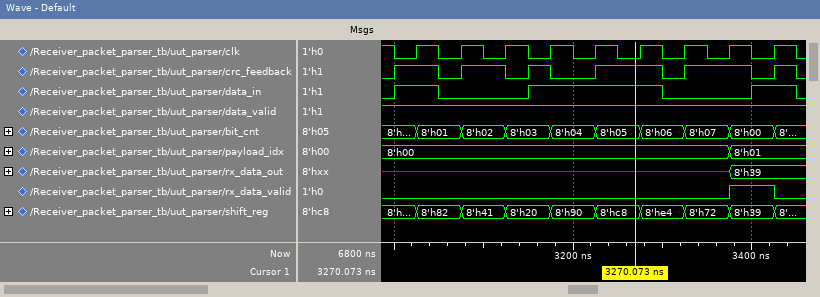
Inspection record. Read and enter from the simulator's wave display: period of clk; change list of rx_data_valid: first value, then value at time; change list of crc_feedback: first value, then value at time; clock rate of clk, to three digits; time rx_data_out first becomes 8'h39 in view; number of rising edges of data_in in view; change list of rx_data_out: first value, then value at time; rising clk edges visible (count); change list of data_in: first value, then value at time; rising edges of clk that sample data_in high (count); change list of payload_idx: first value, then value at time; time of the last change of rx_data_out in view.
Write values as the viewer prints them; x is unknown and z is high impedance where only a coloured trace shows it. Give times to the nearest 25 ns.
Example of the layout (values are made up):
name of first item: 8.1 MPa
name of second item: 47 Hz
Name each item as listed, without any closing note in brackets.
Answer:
period of clk: 50 ns
change list of rx_data_valid: first value, then value at time: 0, 1 at 3375 ns, 0 at 3425 ns
change list of crc_feedback: first value, then value at time: 0, 1 at 3000 ns, 0 at 3050 ns, 1 at 3075 ns, 0 at 3125 ns, 1 at 3150 ns, 0 at 3175 ns, 1 at 3225 ns, 0 at 3300 ns, 1 at 3325 ns, 0 at 3400 ns, 1 at 3425 ns, 0 at 3450 ns
clock rate of clk, to three digits: 20.0 MHz
time rx_data_out first becomes 8'h39 in view: 3375 ns
number of rising edges of data_in in view: 3
change list of rx_data_out: first value, then value at time: x, 8'h39 at 3375 ns
rising clk edges visible: 9
change list of data_in: first value, then value at time: 0, 1 at 3000 ns, 0 at 3050 ns, 1 at 3150 ns, 0 at 3300 ns, 1 at 3400 ns, 0 at 3450 ns
rising edges of clk that sample data_in high: 5
change list of payload_idx: first value, then value at time: 8'h00, 8'h01 at 3375 ns
time of the last change of rx_data_out in view: 3375 ns
